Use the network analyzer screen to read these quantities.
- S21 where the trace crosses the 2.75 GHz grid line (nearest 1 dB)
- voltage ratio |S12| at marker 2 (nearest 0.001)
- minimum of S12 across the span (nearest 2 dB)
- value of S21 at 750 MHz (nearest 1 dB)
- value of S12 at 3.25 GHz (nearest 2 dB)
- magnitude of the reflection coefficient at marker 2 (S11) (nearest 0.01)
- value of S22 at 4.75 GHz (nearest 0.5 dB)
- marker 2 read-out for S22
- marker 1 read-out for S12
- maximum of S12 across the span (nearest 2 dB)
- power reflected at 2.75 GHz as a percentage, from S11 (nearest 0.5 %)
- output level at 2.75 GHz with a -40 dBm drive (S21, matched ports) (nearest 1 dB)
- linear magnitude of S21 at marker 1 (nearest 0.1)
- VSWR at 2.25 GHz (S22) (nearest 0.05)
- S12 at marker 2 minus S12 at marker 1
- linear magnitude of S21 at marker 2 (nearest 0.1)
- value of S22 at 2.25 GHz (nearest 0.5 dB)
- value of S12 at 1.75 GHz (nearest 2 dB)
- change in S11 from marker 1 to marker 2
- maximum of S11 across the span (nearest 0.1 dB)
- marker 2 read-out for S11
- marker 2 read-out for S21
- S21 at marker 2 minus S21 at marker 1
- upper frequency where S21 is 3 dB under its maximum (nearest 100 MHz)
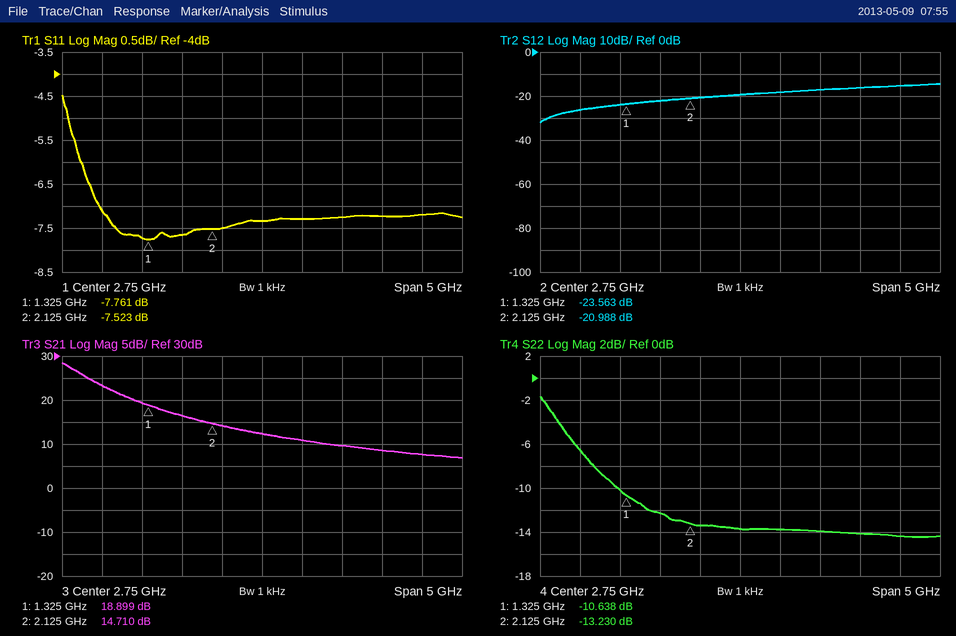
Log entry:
12 dB
0.089
-32 dB
23 dB
-18 dB
0.42
-14.5 dB
-13.230 dB
-23.563 dB
-14 dB
18.5 %
-28 dBm
8.8
1.55
2.575 dB
5.4
-13.5 dB
-22 dB
0.238 dB
-4.5 dB
-7.523 dB
14.710 dB
-4.189 dB
500 MHz
